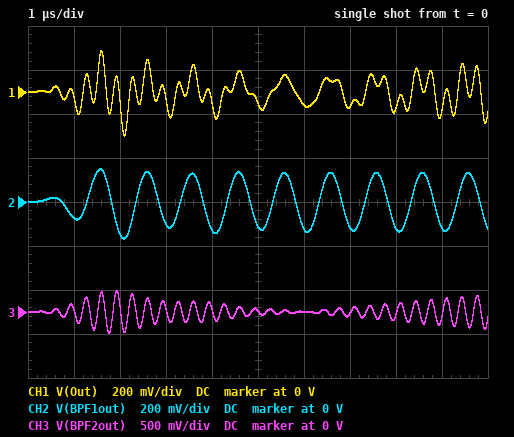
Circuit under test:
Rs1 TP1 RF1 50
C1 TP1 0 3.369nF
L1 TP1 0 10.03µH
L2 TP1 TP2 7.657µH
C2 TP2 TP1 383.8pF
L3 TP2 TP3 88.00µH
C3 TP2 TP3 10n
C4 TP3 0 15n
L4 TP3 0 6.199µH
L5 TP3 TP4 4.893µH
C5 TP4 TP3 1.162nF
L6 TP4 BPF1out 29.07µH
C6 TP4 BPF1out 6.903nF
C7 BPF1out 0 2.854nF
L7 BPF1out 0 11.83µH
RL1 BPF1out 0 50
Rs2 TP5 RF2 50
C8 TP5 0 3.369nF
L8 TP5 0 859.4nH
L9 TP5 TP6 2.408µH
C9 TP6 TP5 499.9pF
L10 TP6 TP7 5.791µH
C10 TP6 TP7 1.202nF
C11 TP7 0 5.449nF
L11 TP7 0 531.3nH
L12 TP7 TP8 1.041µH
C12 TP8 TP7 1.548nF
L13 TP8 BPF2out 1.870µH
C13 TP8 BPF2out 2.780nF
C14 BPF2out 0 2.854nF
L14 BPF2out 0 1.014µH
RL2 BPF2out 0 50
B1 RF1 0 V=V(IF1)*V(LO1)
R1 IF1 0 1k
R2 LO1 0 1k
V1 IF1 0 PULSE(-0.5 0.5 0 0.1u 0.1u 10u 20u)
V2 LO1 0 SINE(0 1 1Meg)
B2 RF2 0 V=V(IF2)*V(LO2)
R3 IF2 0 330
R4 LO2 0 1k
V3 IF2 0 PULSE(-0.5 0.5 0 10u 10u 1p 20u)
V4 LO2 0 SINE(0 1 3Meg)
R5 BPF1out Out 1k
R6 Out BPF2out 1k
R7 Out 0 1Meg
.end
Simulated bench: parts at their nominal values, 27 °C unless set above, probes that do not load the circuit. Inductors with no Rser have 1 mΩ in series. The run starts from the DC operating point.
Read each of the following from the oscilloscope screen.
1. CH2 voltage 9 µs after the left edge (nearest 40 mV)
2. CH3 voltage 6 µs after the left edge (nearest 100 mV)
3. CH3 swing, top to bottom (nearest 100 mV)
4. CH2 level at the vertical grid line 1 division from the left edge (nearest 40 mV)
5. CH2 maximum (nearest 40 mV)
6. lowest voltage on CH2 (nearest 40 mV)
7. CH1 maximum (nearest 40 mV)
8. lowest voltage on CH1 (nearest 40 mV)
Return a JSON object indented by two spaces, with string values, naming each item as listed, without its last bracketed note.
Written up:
{
  "CH2 voltage 9 µs after the left edge": "-120 mV",
  "CH3 voltage 6 µs after the left edge": "0 V",
  "CH3 swing, top to bottom": "500 mV",
  "CH2 level at the vertical grid line 1 division from the left edge": "-80 mV",
  "CH2 maximum": "160 mV",
  "lowest voltage on CH2": "-160 mV",
  "CH1 maximum": "200 mV",
  "lowest voltage on CH1": "-200 mV"
}
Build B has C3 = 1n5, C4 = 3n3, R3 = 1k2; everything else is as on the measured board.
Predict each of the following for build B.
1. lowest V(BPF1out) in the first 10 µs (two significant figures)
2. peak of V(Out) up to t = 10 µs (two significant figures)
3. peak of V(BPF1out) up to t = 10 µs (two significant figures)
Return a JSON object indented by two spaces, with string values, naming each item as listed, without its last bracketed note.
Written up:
{
  "lowest V(BPF1out) in the first 10 µs": "-190 mV",
  "peak of V(Out) up to t = 10 µs": "180 mV",
  "peak of V(BPF1out) up to t = 10 µs": "190 mV"
}
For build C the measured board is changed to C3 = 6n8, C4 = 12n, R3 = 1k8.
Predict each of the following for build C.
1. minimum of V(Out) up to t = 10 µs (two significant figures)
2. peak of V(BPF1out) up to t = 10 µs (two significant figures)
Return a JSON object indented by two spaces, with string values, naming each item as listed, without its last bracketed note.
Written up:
{
  "minimum of V(Out) up to t = 10 µs": "-210 mV",
  "peak of V(BPF1out) up to t = 10 µs": "190 mV"
}
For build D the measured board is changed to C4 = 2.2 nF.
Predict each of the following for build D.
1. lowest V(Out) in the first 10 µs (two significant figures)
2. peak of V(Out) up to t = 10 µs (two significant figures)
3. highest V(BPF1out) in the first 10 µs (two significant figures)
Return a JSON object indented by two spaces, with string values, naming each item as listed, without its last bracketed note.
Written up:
{
  "lowest V(Out) in the first 10 µs": "-220 mV",
  "peak of V(Out) up to t = 10 µs": "200 mV",
  "highest V(BPF1out) in the first 10 µs": "220 mV"
}
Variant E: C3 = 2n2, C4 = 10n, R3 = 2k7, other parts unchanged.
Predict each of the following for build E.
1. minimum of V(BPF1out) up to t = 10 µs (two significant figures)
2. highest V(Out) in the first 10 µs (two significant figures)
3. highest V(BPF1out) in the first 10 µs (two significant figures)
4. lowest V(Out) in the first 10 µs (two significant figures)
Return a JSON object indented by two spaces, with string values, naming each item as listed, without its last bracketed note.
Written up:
{
  "minimum of V(BPF1out) up to t = 10 µs": "-170 mV",
  "highest V(Out) in the first 10 µs": "170 mV",
  "highest V(BPF1out) in the first 10 µs": "160 mV",
  "lowest V(Out) in the first 10 µs": "-190 mV"
}
